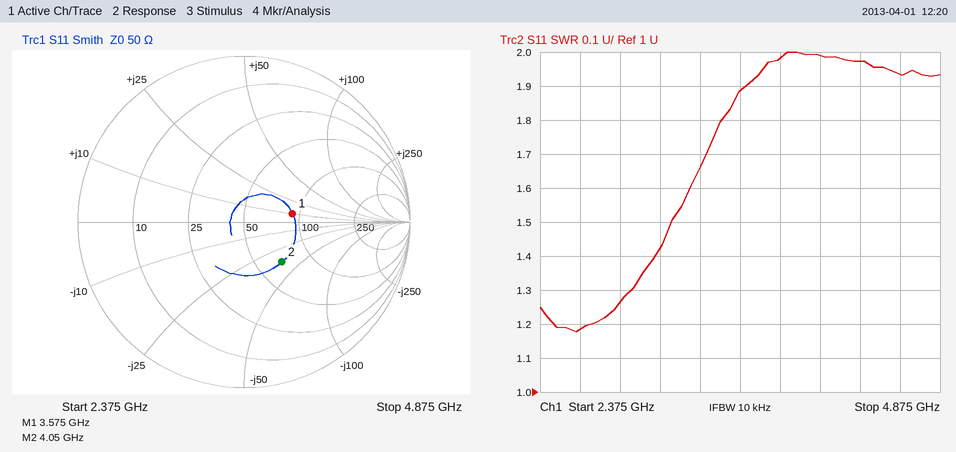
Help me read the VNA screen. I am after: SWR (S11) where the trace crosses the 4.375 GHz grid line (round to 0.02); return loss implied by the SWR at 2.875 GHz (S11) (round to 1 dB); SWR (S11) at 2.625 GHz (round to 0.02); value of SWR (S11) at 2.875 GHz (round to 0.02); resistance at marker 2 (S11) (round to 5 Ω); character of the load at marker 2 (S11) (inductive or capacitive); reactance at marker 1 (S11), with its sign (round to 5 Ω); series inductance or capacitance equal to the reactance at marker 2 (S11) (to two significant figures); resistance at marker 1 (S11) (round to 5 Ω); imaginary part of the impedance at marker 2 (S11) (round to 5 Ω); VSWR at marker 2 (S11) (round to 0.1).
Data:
1.98
19 dB
1.18
1.26
70 Ω
capacitive
+10 Ω
1.1 pF
90 Ω
-35 Ω
2.0
